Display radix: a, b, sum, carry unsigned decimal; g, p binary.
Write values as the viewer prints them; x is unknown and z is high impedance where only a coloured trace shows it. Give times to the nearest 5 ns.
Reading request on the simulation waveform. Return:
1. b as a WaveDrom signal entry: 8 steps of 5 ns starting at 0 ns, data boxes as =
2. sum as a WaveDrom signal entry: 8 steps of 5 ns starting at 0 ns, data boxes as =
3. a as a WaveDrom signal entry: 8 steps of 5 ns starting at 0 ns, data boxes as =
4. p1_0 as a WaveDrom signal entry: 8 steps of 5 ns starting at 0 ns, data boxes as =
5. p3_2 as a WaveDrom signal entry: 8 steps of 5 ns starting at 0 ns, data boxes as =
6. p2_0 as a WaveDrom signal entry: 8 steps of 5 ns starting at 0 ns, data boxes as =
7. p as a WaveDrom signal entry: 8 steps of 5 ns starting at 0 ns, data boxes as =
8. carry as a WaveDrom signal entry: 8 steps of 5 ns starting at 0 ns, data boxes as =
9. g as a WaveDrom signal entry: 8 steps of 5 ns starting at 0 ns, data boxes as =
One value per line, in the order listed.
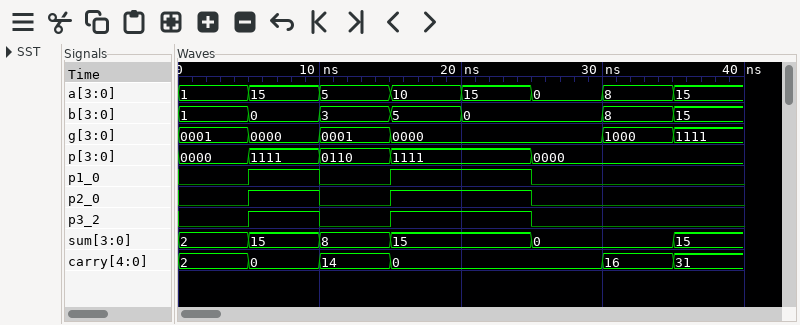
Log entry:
{name: 'b', wave: '=====.==', data: '1 0 3 5 0 8 15'}
{name: 'sum', wave: '====.=.=', data: '2 15 8 15 0 15'}
{name: 'a', wave: '========', data: '1 15 5 10 15 0 8 15'}
{name: 'p1_0', wave: '0101.0..'}
{name: 'p3_2', wave: '0101.0..'}
{name: 'p2_0', wave: '0101.0..'}
{name: 'p', wave: '====.=..', data: '0000 1111 0110 1111 0000'}
{name: 'carry', wave: '====..==', data: '2 0 14 0 16 31'}
{name: 'g', wave: '====..==', data: '0001 0000 0001 0000 1000 1111'}
